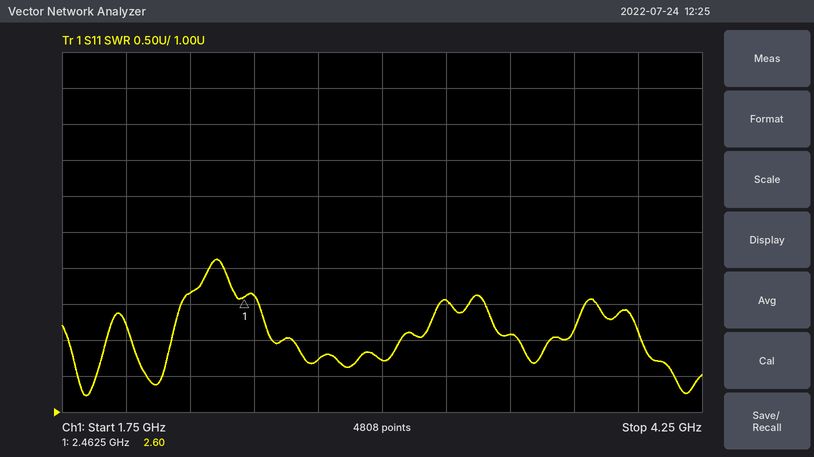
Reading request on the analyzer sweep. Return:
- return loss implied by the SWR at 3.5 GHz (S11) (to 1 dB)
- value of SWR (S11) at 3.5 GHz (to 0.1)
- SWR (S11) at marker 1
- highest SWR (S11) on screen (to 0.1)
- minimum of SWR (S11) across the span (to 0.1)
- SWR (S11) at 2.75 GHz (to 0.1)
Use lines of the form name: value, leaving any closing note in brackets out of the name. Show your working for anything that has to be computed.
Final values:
return loss implied by the SWR at 3.5 GHz (S11): −20 log10((2.1 − 1)/(2.1 + 1)) ≈ 9 dB
value of SWR (S11) at 3.5 GHz: 2.1
SWR (S11) at marker 1: 2.60
highest SWR (S11) on screen: 3.1
minimum of SWR (S11) across the span: 1.2
SWR (S11) at 2.75 GHz: 1.7
